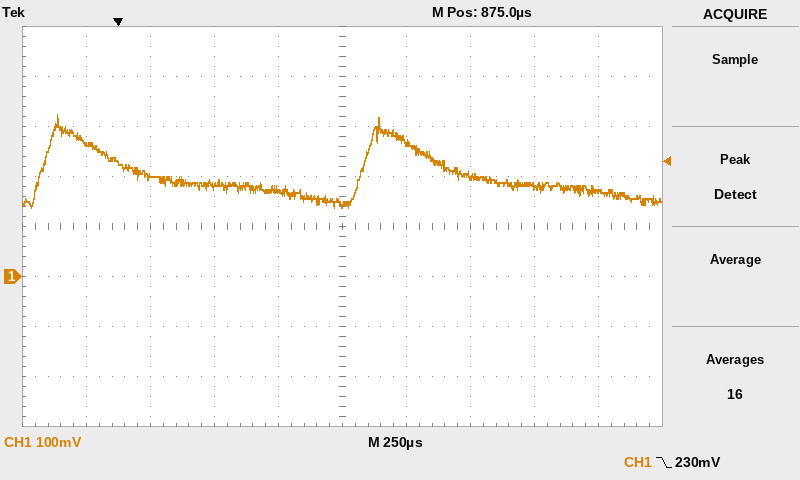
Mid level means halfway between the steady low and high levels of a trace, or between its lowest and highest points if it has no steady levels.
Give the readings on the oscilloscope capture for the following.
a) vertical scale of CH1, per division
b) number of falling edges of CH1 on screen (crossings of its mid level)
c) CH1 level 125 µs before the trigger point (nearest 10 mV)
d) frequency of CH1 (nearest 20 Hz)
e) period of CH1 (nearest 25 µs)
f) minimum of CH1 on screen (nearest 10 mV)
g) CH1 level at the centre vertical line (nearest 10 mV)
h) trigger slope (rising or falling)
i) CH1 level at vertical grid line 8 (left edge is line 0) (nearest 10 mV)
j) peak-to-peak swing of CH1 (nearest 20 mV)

100 mV
2
270 mV
800 Hz
1.250 ms
140 mV
140 mV
falling
180 mV
180 mV
